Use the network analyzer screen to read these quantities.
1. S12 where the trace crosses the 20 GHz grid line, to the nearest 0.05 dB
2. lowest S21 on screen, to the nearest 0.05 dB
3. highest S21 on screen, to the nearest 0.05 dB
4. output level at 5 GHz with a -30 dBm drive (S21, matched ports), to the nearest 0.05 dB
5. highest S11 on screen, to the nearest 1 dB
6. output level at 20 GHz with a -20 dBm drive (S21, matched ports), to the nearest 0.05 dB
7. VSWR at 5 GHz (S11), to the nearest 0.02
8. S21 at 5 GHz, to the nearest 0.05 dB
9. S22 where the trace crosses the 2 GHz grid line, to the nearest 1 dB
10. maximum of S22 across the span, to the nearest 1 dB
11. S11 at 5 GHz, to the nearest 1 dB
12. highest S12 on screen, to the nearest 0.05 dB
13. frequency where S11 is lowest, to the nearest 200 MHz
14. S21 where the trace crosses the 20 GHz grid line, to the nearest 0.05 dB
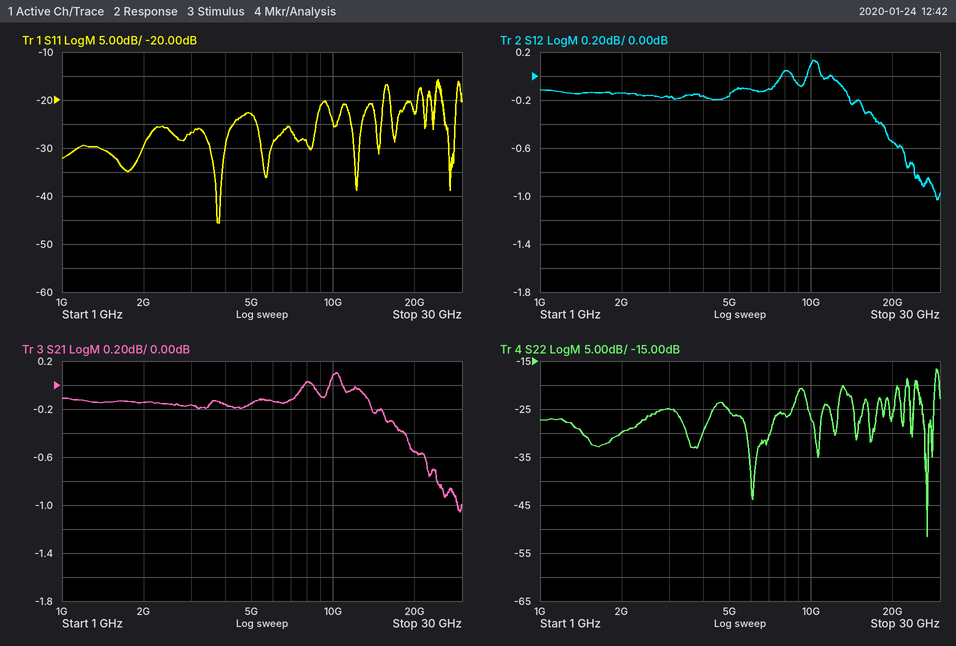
-0.55 dB
-1.05 dB
0.10 dB
-30.15 dBm
-16 dB
-20.55 dBm
1.16
-0.15 dB
-30 dB
-17 dB
-23 dB
0.15 dB
3.8 GHz
-0.55 dB
